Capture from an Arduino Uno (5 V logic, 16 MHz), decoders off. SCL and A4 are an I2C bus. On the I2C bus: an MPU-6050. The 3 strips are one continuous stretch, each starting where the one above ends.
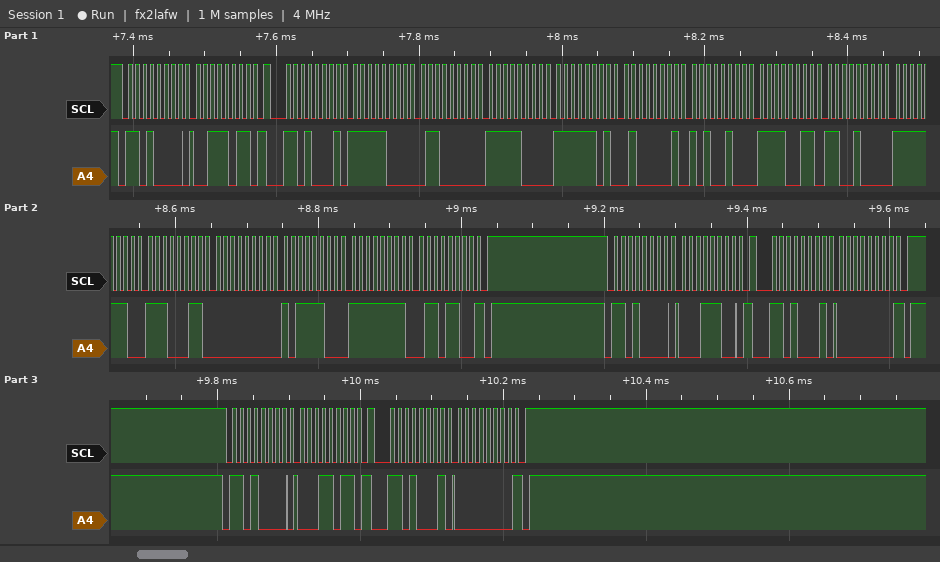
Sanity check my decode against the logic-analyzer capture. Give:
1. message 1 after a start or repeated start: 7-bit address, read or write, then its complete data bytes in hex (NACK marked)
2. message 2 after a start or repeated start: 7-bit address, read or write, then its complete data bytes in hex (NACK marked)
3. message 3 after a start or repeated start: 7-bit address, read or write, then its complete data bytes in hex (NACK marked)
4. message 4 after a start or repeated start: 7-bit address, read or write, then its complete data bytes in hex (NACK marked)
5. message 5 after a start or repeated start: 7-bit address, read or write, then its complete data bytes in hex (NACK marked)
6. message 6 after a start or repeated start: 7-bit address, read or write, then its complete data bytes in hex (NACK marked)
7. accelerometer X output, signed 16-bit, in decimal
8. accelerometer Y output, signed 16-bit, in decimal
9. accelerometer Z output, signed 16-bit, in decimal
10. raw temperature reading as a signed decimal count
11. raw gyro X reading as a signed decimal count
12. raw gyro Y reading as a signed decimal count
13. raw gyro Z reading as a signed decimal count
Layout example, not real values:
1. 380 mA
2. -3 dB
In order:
1. 0x68 write: 3B
2. 0x68 read: F8 60 F8 FD 41 A4 F3 C8 FE E3 00 BC FF 6C NACK
3. 0x68 write: 1C
4. 0x68 read: 00 NACK
5. 0x68 write: 1B
6. 0x68 read: 00 NACK
7. -1952
8. -1795
9. 16804
10. -3128
11. -285
12. 188
13. -148
